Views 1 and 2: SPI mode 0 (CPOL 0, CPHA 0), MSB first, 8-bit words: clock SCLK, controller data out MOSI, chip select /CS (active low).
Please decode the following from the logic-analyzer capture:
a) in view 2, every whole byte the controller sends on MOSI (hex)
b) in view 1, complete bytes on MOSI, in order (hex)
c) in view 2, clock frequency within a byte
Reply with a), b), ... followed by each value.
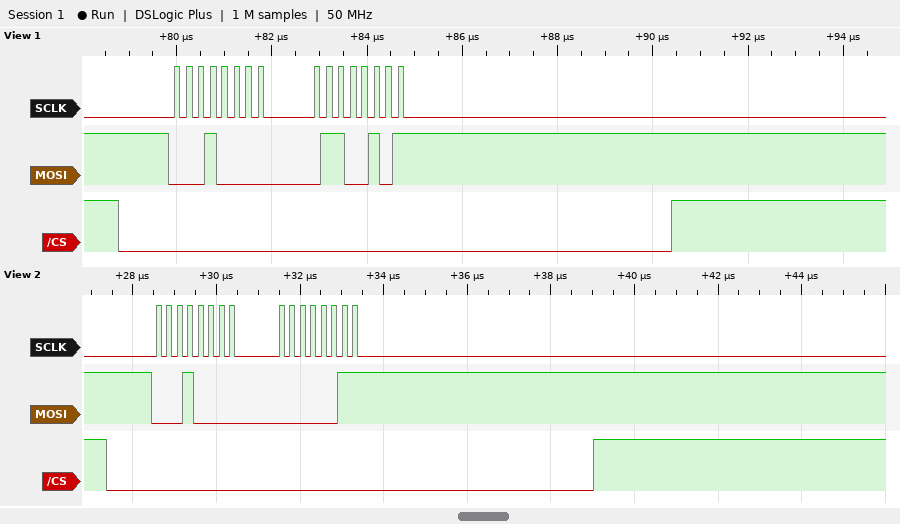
a) 10 03
b) 10 65
c) 4 MHz
